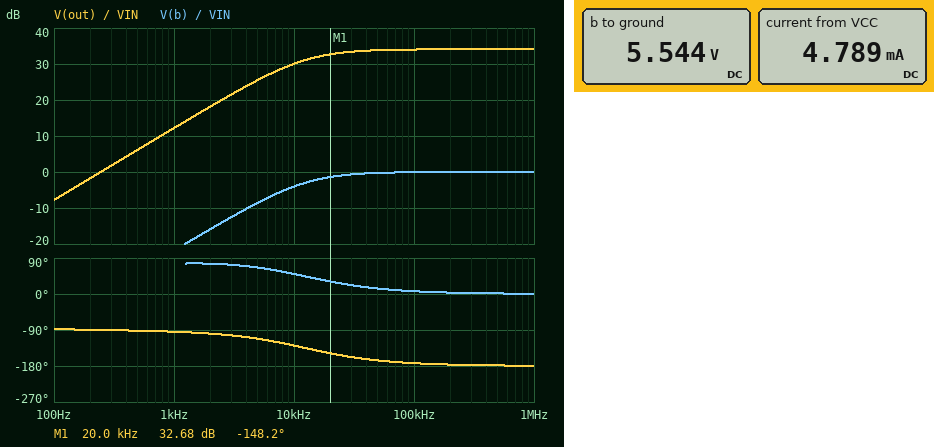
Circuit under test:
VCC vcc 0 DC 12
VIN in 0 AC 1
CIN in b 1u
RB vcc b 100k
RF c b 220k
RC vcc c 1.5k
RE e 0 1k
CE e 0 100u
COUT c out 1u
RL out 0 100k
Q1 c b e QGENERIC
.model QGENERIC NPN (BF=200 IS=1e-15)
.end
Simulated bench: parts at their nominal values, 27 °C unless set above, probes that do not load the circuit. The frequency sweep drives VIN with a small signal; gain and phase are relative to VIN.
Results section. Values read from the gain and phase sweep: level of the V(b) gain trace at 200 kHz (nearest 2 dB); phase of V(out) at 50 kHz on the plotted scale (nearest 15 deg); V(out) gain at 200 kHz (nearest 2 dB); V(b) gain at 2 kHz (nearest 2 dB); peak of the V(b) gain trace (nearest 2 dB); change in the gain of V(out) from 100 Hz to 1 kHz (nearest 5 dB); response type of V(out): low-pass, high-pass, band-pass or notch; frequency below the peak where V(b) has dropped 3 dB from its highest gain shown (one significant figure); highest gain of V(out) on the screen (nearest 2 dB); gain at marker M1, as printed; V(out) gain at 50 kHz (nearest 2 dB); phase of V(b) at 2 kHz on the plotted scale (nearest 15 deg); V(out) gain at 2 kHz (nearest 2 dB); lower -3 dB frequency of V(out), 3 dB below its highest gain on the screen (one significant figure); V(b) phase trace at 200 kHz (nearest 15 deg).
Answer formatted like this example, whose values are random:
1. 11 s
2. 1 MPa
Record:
1. 0 dB
2. -165 deg
3. 34 dB
4. -16 dB
5. 0 dB
6. 20 dB
7. high-pass
8. 10 kHz
9. 34 dB
10. 32.68 dB
11. 34 dB
12. 75 deg
13. 18 dB
14. 10 kHz
15. 0 deg
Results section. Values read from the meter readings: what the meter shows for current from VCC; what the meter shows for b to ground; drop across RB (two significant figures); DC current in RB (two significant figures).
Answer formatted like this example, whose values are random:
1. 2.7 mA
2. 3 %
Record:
1. 4.789 mA
2. 5.544 V
3. 6.5 V
4. 65 µA
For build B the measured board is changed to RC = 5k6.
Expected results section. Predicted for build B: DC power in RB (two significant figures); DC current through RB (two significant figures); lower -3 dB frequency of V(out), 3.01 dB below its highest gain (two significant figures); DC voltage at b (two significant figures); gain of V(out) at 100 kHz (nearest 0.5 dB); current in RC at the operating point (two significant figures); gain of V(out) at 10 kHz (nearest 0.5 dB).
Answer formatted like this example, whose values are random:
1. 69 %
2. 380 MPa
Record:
1. 880 µW
2. 94 µA
3. 6.0 kHz
4. 2.6 V
5. 20.5 dB
6. 1.8 mA
7. 19.5 dB
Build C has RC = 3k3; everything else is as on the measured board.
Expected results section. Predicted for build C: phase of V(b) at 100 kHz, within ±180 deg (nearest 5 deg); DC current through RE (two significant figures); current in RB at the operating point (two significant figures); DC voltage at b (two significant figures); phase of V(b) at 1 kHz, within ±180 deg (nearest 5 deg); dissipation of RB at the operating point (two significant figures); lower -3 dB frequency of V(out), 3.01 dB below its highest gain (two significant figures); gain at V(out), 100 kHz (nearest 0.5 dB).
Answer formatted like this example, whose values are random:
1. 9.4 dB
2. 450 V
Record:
1. 5 deg
2. 2.8 mA
3. 84 µA
4. 3.6 V
5. 80 deg
6. 710 µW
7. 8.6 kHz
8. 25.5 dB
